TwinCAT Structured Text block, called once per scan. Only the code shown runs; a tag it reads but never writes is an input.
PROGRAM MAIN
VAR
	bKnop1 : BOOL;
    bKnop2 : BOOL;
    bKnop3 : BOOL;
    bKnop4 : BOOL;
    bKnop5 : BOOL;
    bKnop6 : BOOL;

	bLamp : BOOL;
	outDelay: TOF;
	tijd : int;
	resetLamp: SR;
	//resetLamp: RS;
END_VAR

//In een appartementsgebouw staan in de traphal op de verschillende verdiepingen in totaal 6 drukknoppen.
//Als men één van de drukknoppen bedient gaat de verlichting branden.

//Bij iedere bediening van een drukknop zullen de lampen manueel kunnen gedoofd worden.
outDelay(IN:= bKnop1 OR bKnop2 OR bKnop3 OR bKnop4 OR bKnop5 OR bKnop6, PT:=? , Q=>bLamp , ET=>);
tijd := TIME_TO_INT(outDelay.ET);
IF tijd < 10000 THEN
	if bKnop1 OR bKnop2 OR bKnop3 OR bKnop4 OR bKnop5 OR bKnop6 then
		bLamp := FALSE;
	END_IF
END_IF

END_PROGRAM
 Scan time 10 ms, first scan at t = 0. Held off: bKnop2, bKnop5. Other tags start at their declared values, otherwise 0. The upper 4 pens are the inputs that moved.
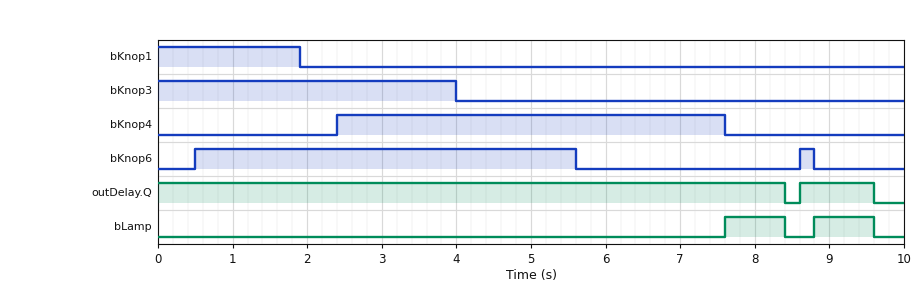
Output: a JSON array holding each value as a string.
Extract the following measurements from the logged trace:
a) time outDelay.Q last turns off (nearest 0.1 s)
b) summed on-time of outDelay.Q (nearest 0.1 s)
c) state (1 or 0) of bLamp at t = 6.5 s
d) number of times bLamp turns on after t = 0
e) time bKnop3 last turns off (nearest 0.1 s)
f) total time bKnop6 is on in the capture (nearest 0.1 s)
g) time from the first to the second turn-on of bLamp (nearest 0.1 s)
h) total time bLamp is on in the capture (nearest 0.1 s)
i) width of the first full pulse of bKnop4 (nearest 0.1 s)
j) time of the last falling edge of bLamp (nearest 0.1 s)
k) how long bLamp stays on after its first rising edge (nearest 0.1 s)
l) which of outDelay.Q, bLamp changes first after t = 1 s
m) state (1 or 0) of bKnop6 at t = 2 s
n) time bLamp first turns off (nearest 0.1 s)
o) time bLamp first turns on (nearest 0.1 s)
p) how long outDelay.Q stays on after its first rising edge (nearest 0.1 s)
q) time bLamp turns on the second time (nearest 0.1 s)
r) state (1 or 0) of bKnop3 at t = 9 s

["9.6 s", "9.4 s", "0", "2", "4.0 s", "5.3 s", "1.2 s", "1.6 s", "5.2 s", "9.6 s", "0.8 s", "bLamp", "1", "8.4 s", "7.6 s", "1.0 s", "8.8 s", "0"]
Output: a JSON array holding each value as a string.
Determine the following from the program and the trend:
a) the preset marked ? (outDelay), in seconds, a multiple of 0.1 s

["0.8 s"]
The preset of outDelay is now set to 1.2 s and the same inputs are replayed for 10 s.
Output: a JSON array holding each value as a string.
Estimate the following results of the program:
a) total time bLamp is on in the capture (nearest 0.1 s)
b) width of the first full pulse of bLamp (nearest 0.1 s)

["2.2 s", "1.0 s"]
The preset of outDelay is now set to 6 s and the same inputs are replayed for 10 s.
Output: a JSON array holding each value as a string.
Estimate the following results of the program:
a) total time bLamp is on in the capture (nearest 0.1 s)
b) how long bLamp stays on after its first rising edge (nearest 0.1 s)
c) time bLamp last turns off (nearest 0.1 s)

["2.2 s", "1.0 s", "8.6 s"]
